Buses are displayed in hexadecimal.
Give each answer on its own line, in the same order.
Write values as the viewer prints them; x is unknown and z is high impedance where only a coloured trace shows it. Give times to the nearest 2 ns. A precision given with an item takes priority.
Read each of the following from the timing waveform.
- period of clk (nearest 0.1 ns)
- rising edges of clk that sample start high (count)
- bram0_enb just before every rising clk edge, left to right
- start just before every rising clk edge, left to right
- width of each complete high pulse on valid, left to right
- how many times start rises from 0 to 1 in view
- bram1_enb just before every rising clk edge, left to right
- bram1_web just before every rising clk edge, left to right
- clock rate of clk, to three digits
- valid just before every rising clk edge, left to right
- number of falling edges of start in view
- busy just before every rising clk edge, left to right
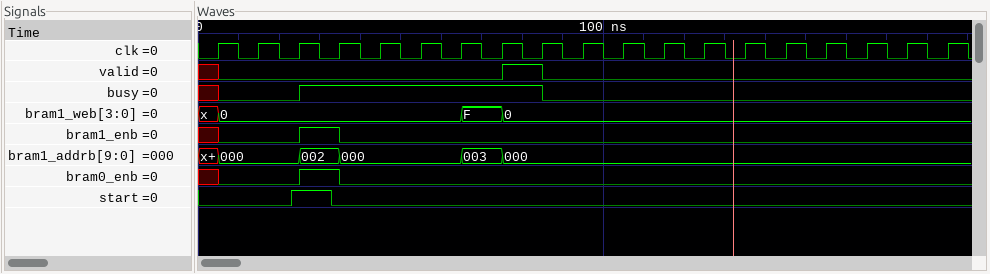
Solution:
10 ns
1
x 0 0 1 0 0 0 0 0 0 0 0 0 0 0 0 0 0 0
0 0 1 0 0 0 0 0 0 0 0 0 0 0 0 0 0 0 0
10 ns
1
x 0 0 1 0 0 0 0 0 0 0 0 0 0 0 0 0 0 0
x, 0, 0, 0, 0, 0, 0, F, 0, 0, 0, 0, 0, 0, 0, 0, 0, 0, 0
100 MHz
x 0 0 0 0 0 0 0 1 0 0 0 0 0 0 0 0 0 0
1
x 0 0 1 1 1 1 1 1 0 0 0 0 0 0 0 0 0 0
